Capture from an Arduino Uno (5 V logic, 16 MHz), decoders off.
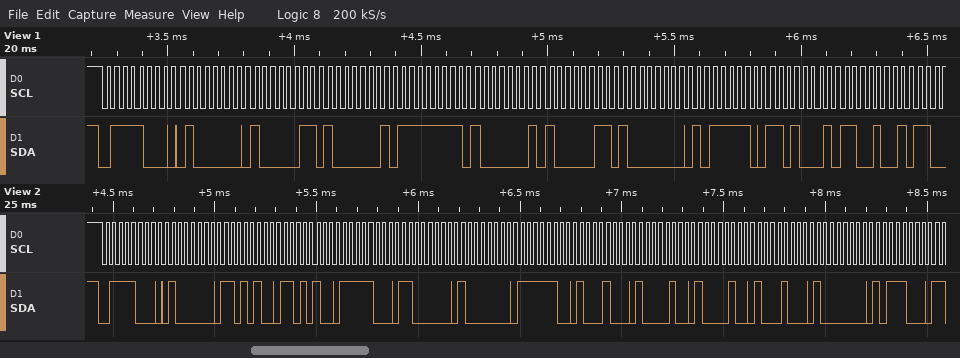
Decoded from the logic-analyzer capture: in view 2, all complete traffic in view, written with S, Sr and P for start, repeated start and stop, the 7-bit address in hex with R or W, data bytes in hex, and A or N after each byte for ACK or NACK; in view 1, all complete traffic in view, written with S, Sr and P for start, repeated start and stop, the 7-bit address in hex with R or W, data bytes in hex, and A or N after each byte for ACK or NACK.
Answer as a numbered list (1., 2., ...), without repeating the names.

1. S 3CW A 40 A D4 A D4 A F8 A C0 A 80 A FC A 88 A 84 A 84 A 88 A 80 A B8 A
2. S 3CW A 40 A 83 A 81 A FF A 81 A 83 A 80 A BE A D1 A C9 A
